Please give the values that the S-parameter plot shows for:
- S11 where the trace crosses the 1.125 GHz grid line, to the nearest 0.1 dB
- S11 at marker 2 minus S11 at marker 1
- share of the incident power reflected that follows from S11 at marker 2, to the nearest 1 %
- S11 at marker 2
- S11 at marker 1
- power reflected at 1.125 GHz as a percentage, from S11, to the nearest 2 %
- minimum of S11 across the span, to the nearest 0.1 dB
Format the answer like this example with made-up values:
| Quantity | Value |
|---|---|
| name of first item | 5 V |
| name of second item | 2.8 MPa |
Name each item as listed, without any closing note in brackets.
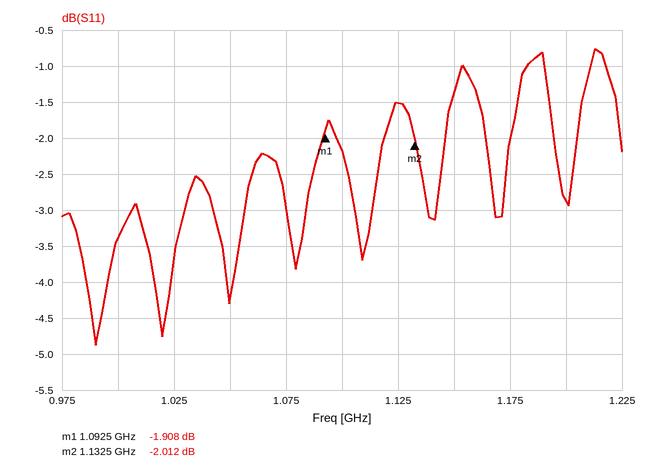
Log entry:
| Quantity | Value |
|---|---|
| S11 where the trace crosses the 1.125 GHz grid line, to the nearest 0.1 dB | -1.5 dB |
| S11 at marker 2 minus S11 at marker 1 | -0.104 dB |
| share of the incident power reflected that follows from S11 at marker 2, to the nearest 1 % | 63 % |
| S11 at marker 2 | -2.012 dB |
| S11 at marker 1 | -1.908 dB |
| power reflected at 1.125 GHz as a percentage, from S11, to the nearest 2 % | 70 % |
| minimum of S11 across the span, to the nearest 0.1 dB | -4.9 dB |
